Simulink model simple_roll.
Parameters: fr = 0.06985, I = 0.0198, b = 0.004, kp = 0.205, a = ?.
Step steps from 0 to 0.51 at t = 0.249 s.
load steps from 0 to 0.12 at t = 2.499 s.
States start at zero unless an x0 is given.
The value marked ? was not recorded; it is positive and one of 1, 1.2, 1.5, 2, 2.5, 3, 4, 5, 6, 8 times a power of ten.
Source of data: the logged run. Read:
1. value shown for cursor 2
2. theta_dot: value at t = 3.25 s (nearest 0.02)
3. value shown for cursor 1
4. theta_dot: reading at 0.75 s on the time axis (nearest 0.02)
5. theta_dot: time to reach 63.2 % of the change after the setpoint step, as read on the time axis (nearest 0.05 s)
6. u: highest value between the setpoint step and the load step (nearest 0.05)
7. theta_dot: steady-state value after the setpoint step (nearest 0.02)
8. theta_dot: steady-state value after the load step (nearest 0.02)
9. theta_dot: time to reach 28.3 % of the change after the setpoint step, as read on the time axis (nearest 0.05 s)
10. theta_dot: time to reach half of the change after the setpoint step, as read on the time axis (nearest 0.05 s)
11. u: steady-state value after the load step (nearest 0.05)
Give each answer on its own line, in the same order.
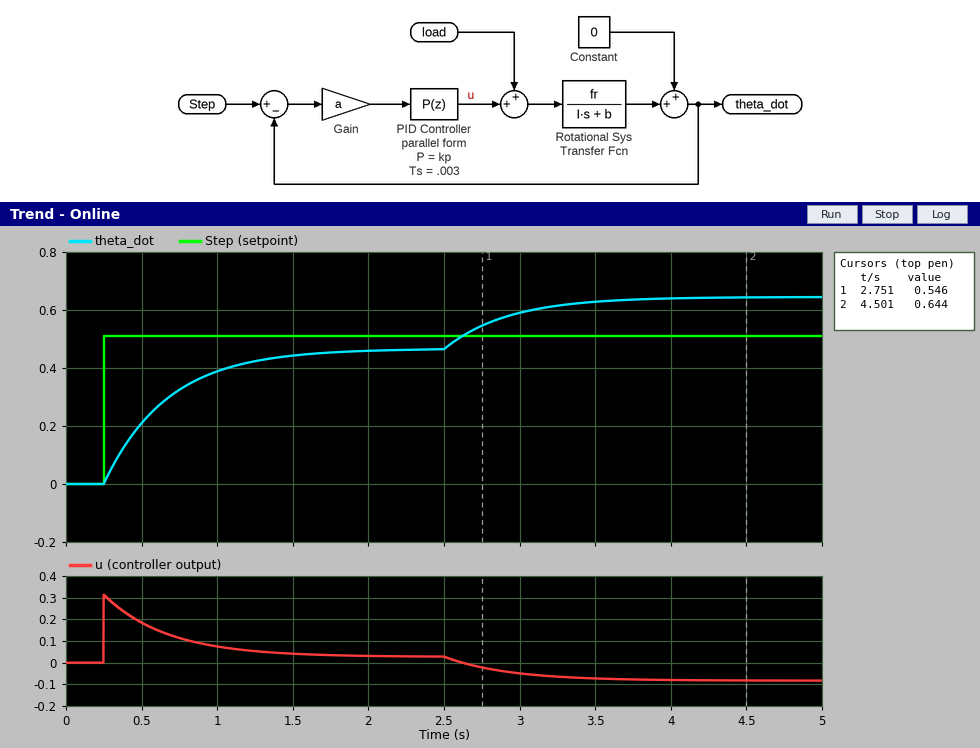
0.644
0.62
0.546
0.32
0.65 s
0.30
0.46
0.64
0.40 s
0.55 s
-0.10
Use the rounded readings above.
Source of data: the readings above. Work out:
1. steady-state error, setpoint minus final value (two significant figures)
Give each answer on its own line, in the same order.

0.050
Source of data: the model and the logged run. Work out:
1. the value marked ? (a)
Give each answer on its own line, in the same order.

3
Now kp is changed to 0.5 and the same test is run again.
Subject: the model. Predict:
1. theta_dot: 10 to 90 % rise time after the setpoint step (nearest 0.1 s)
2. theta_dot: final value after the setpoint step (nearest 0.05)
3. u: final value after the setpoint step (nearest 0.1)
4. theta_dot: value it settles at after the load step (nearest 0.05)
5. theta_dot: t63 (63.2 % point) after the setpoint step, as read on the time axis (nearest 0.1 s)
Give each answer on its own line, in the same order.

0.4 s
0.50
0.0
0.55
0.4 s
